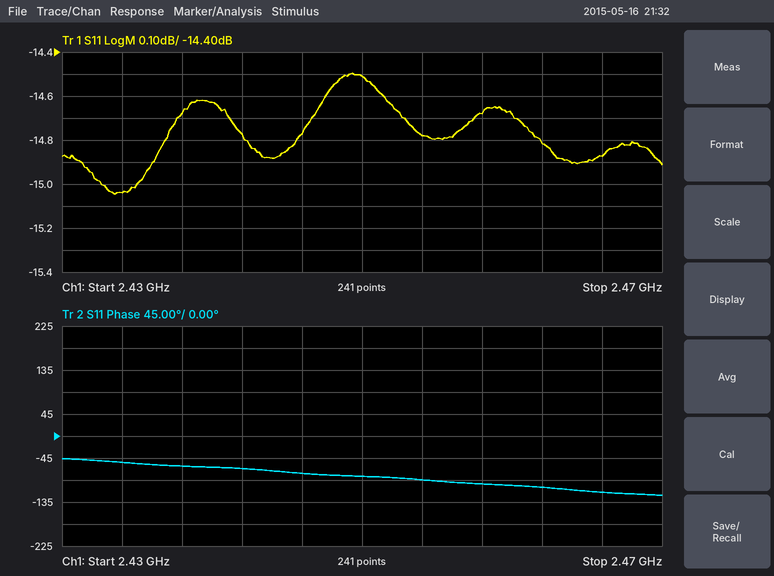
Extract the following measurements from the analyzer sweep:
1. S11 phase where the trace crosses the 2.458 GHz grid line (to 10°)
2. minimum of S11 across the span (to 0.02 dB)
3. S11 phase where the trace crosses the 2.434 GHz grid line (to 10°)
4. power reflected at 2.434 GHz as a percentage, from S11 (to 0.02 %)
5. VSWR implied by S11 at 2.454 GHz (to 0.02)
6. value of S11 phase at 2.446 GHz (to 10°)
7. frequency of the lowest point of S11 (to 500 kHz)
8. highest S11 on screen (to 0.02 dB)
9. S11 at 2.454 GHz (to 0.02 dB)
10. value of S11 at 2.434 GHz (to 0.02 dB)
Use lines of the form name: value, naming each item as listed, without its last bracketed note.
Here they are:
S11 phase where the trace crosses the 2.458 GHz grid line: -100°
minimum of S11 across the span: -15.04 dB
S11 phase where the trace crosses the 2.434 GHz grid line: -50°
power reflected at 2.434 GHz as a percentage, from S11: 3.14 %
VSWR implied by S11 at 2.454 GHz: 1.44
value of S11 phase at 2.446 GHz: -80°
frequency of the lowest point of S11: 2.4335 GHz
highest S11 on screen: -14.50 dB
S11 at 2.454 GHz: -14.78 dB
value of S11 at 2.434 GHz: -15.04 dB
